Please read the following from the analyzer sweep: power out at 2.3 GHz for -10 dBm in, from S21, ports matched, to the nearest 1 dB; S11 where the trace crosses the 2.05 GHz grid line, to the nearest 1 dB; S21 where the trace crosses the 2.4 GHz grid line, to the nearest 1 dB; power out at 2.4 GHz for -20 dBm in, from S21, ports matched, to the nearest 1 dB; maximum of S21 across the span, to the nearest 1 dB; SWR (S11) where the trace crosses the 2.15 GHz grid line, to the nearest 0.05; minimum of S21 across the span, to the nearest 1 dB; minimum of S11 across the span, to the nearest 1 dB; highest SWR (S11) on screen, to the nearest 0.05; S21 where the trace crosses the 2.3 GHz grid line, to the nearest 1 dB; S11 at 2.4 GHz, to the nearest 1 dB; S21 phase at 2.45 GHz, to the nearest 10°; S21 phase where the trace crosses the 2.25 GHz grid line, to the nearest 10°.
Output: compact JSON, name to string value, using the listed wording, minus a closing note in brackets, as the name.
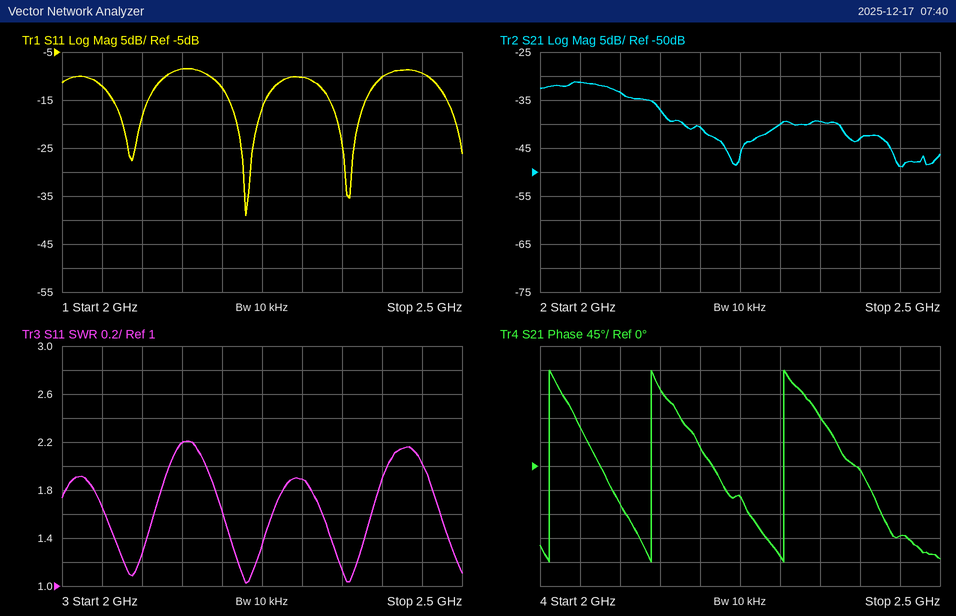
{"power out at 2.3 GHz for -10 dBm in, from S21, ports matched, to the nearest 1 dB": "-50 dBm", "S11 where the trace crosses the 2.05 GHz grid line, to the nearest 1 dB": "-12 dB", "S21 where the trace crosses the 2.4 GHz grid line, to the nearest 1 dB": "-43 dB", "power out at 2.4 GHz for -20 dBm in, from S21, ports matched, to the nearest 1 dB": "-63 dBm", "maximum of S21 across the span, to the nearest 1 dB": "-31 dB", "SWR (S11) where the trace crosses the 2.15 GHz grid line, to the nearest 0.05": "2.20", "minimum of S21 across the span, to the nearest 1 dB": "-49 dB", "minimum of S11 across the span, to the nearest 1 dB": "-39 dB", "highest SWR (S11) on screen, to the nearest 0.05": "2.20", "S21 where the trace crosses the 2.3 GHz grid line, to the nearest 1 dB": "-40 dB", "S11 at 2.4 GHz, to the nearest 1 dB": "-10 dB", "S21 phase at 2.45 GHz, to the nearest 10°": "-130°", "S21 phase where the trace crosses the 2.25 GHz grid line, to the nearest 10°": "-60°"}
